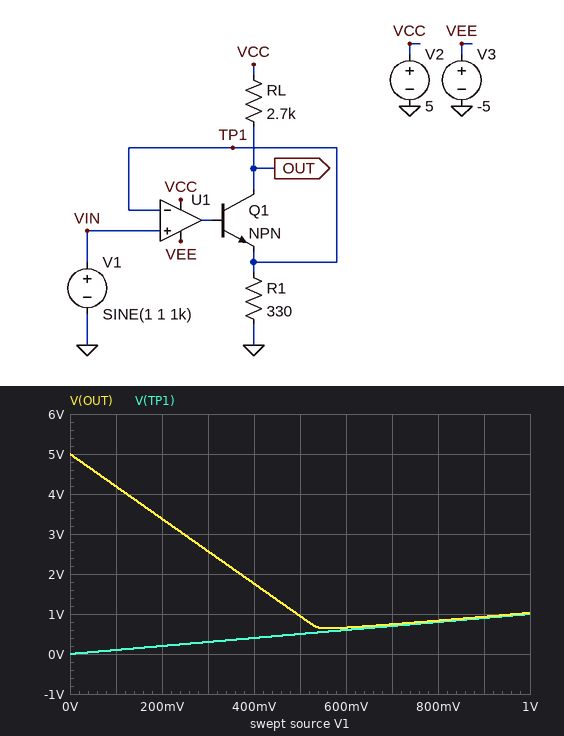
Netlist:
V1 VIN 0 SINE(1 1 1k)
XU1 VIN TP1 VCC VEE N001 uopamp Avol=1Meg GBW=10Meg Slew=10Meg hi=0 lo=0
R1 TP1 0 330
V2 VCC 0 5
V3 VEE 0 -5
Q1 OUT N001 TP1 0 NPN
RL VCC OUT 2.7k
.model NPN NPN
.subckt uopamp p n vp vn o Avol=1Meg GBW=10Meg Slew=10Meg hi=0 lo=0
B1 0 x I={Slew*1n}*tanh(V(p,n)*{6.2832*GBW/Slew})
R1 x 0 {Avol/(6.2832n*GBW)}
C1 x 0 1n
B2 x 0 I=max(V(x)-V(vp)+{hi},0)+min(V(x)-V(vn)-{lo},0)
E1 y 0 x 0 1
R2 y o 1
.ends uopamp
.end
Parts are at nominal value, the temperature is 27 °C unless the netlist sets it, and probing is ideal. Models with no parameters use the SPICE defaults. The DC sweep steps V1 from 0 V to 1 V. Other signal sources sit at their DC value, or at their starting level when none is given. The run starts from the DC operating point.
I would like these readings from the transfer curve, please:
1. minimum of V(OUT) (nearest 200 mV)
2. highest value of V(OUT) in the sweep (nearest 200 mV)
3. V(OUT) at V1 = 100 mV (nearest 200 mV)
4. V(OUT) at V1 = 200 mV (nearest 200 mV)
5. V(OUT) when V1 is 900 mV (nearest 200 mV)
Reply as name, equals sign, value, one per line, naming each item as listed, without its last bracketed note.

minimum of V(OUT) = 600 mV
highest value of V(OUT) in the sweep = 5.0 V
V(OUT) at V1 = 100 mV = 4.2 V
V(OUT) at V1 = 200 mV = 3.4 V
V(OUT) when V1 is 900 mV = 1.0 V
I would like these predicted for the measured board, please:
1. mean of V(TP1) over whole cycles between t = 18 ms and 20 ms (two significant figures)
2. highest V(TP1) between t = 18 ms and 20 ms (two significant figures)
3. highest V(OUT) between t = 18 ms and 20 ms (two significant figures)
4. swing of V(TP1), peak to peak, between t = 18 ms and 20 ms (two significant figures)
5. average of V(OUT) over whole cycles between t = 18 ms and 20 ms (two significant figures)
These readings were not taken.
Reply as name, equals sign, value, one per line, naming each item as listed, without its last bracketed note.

mean of V(TP1) over whole cycles between t = 18 ms and 20 ms = 1.0 V
highest V(TP1) between t = 18 ms and 20 ms = 2.0 V
highest V(OUT) between t = 18 ms and 20 ms = 5.0 V
swing of V(TP1), peak to peak, between t = 18 ms and 20 ms = 2.0 V
average of V(OUT) over whole cycles between t = 18 ms and 20 ms = 2.2 V
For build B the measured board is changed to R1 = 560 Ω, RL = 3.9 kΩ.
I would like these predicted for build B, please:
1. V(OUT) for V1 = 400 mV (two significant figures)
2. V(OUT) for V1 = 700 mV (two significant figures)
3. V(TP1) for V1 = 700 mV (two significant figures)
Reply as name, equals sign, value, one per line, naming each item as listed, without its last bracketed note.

V(OUT) for V1 = 400 mV = 2.2 V
V(OUT) for V1 = 700 mV = 760 mV
V(TP1) for V1 = 700 mV = 700 mV
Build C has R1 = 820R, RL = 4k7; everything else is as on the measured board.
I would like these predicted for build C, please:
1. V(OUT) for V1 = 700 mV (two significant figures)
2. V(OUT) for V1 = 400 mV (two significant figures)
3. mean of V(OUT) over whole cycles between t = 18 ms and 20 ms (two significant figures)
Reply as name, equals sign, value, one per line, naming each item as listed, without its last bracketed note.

V(OUT) for V1 = 700 mV = 1.0 V
V(OUT) for V1 = 400 mV = 2.7 V
mean of V(OUT) over whole cycles between t = 18 ms and 20 ms = 2.4 V
